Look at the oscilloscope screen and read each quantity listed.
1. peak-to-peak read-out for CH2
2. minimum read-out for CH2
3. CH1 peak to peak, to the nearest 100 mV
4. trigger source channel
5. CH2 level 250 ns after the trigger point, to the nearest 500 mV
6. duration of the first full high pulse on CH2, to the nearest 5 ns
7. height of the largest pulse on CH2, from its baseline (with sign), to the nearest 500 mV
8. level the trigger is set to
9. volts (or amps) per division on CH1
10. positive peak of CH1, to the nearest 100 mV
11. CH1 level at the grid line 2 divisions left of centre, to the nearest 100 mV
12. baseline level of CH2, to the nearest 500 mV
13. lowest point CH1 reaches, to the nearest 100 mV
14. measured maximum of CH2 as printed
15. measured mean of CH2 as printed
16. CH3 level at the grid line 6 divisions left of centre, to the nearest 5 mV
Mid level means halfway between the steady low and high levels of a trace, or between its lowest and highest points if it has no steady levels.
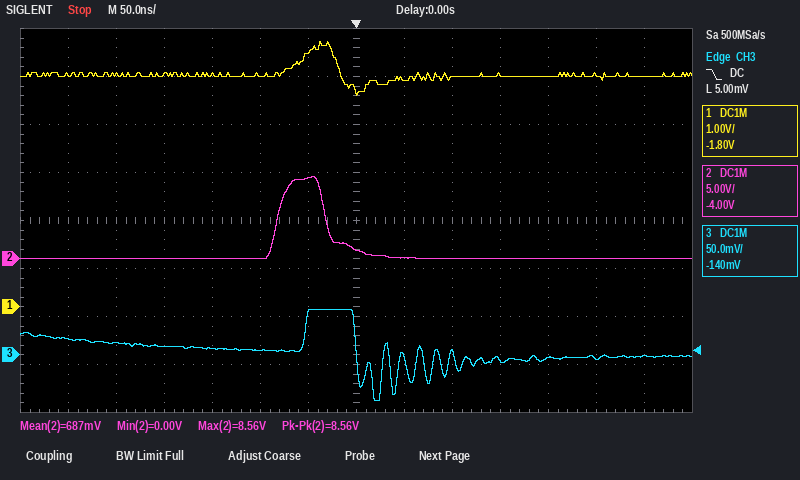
8.56 V
0.00 V
1.1 V
CH3
0.0 V
50 ns
+8.5 V
5.00 mV
1 V
5.5 V
4.8 V
0.0 V
4.4 V
8.56 V
687 mV
15 mV
